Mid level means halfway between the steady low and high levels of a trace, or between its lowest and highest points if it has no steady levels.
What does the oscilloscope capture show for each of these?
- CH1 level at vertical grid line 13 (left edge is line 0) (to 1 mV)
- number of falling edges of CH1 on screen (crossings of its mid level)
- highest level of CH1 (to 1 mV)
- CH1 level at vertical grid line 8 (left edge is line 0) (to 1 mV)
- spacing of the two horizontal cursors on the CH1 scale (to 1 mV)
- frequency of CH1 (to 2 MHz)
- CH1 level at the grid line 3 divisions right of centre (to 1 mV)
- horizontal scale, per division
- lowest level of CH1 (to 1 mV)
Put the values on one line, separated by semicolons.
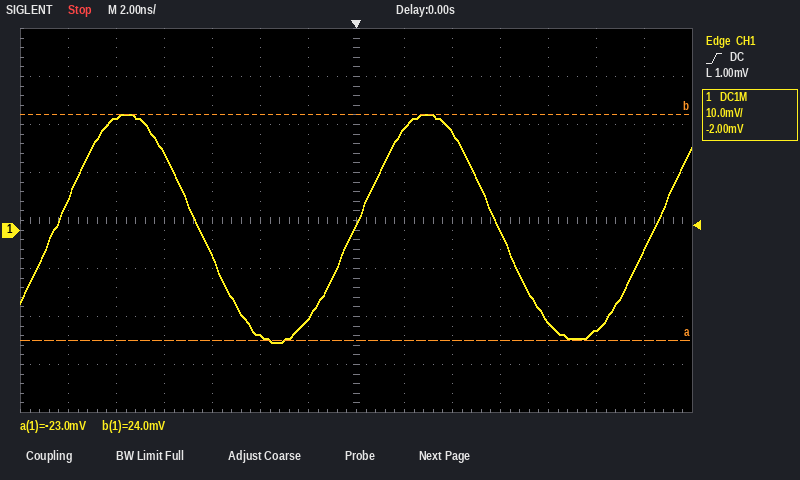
-4 mV; 2; 24 mV; 21 mV; 47 mV; 80 MHz; 0 mV; 2 ns; -23 mV
